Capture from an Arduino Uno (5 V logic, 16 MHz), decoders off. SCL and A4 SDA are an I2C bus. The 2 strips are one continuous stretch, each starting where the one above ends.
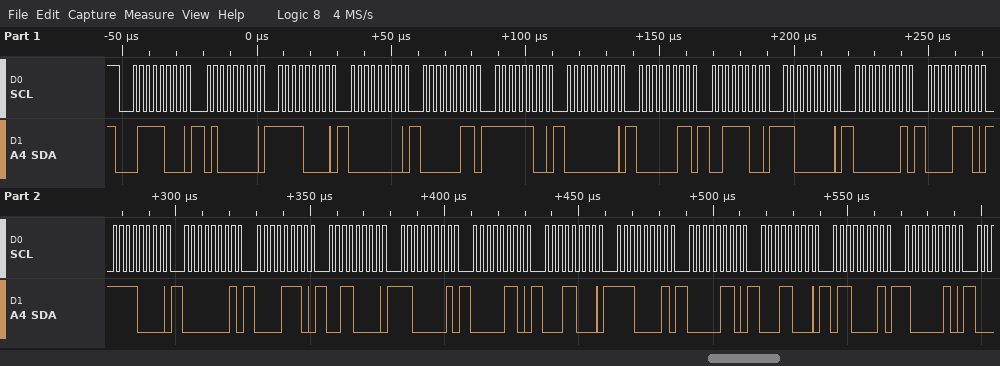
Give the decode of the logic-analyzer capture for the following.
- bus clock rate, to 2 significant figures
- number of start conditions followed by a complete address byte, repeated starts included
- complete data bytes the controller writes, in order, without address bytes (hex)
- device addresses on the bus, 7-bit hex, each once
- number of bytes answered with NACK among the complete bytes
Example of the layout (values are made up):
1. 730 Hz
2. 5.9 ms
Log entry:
1. 400 kHz
2. 1
3. 40 F0 00 03 FC 00 03 3C C0 01 0E F0 01 0E 30 C1 06 18 E1 06 18 61 82
4. 0x3C
5. 0
